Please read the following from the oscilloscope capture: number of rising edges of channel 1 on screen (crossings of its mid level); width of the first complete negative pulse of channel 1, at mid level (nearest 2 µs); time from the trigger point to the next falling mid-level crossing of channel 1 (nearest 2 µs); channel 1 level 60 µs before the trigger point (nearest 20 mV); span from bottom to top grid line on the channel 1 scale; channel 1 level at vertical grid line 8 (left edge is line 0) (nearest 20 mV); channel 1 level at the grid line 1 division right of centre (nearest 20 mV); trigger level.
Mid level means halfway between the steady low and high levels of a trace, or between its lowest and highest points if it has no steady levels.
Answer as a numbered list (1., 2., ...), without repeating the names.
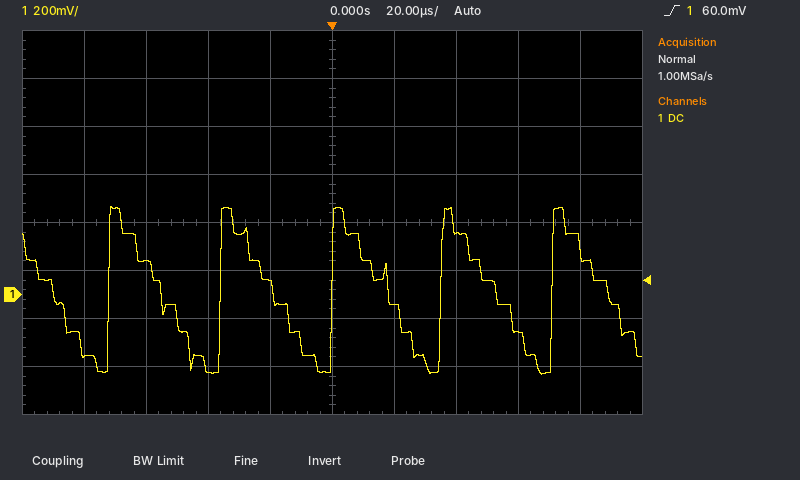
1. 5
2. 18 µs
3. 18 µs
4. 140 mV
5. 1.6 V
6. -160 mV
7. -40 mV
8. 60.0 mV
